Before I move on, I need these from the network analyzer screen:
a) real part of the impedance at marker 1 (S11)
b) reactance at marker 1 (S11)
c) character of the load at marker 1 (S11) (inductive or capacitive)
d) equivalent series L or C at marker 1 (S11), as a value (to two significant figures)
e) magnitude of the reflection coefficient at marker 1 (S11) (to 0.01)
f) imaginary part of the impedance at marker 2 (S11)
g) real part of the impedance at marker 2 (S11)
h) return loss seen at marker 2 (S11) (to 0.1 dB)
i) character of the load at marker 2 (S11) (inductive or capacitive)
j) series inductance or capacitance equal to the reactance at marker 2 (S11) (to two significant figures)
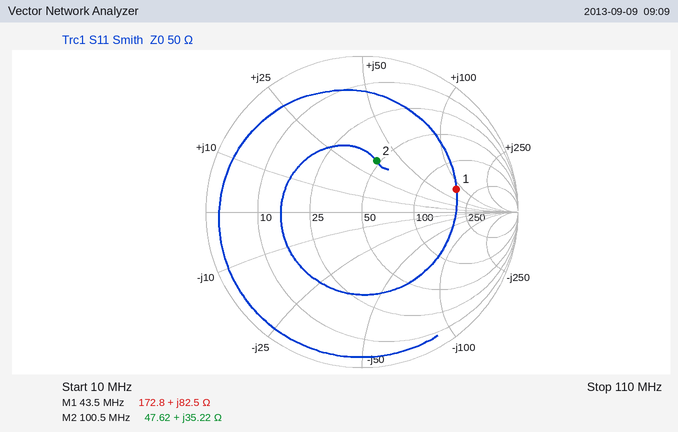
172.8 Ω
+82.5 Ω
inductive
300 nH
0.62
+35.22 Ω
47.62 Ω
9.4 dB
inductive
56 nH
